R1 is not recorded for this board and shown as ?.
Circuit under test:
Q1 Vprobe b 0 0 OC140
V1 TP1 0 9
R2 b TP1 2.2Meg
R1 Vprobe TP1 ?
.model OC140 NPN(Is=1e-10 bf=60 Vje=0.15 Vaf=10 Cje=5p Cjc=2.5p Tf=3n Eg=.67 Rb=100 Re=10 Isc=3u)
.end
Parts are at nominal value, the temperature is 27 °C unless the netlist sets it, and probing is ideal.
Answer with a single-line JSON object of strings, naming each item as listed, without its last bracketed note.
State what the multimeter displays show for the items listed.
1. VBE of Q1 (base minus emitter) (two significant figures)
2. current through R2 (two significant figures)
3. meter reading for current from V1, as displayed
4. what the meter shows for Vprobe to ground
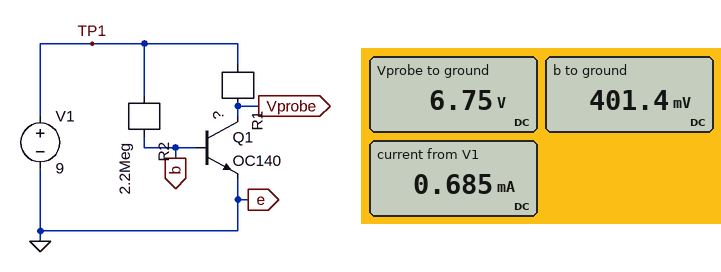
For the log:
{"VBE of Q1 (base minus emitter)": "400 mV", "current through R2": "3.9 µA", "meter reading for current from V1, as displayed": "0.685 mA", "what the meter shows for Vprobe to ground": "6.75 V"}
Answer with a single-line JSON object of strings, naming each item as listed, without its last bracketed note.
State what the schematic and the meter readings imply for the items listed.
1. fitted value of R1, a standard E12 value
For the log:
{"fitted value of R1, a standard E12 value": "3.3 kΩ"}
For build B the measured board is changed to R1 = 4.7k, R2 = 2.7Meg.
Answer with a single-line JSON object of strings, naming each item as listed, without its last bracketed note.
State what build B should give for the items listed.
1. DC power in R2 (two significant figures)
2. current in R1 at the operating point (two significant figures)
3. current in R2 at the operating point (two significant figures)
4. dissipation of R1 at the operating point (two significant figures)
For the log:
{"DC power in R2": "27 µW", "current in R1 at the operating point": "590 µA", "current in R2 at the operating point": "3.2 µA", "dissipation of R1 at the operating point": "1.6 mW"}
